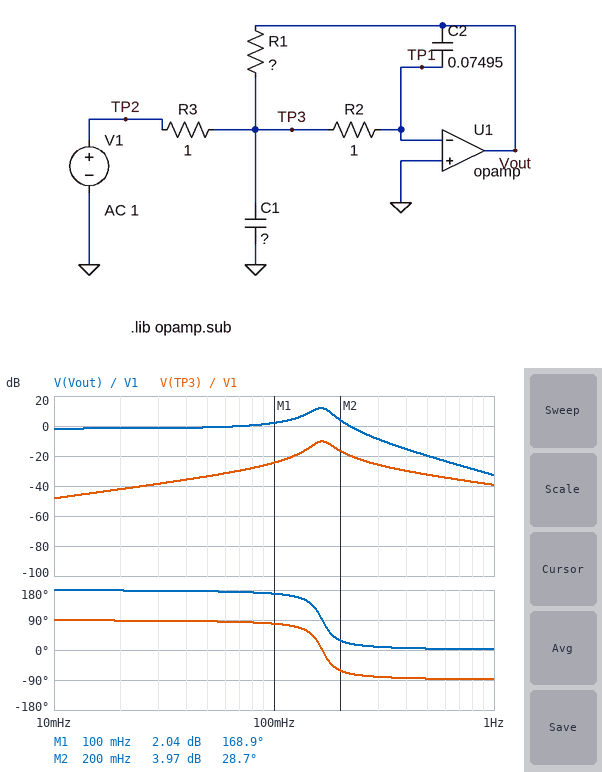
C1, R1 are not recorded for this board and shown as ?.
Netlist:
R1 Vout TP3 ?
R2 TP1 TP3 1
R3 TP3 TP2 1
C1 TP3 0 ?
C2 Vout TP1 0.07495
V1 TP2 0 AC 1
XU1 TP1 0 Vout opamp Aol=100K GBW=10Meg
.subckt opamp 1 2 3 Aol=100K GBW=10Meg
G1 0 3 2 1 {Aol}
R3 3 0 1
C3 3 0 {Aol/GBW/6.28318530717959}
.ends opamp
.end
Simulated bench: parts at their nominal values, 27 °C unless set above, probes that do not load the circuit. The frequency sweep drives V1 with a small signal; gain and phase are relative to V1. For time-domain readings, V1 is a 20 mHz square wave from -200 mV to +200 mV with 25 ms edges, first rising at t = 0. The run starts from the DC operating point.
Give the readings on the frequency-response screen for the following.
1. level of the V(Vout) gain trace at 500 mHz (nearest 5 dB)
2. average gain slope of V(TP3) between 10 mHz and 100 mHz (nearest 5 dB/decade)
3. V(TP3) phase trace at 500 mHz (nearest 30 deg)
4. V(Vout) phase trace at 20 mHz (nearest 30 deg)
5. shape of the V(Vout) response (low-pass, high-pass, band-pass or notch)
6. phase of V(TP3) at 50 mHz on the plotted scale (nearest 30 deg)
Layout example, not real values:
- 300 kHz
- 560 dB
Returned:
- -20 dB
- 25 dB/decade
- -90 deg
- 180 deg
- low-pass
- 90 deg
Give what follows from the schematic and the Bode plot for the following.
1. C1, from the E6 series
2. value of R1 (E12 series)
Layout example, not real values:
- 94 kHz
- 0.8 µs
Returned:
- 15 F
- 0.82 Ω
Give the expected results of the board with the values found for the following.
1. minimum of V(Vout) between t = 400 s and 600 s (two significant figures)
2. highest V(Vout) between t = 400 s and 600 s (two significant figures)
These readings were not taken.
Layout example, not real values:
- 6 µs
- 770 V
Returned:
- -390 mV
- 390 mV
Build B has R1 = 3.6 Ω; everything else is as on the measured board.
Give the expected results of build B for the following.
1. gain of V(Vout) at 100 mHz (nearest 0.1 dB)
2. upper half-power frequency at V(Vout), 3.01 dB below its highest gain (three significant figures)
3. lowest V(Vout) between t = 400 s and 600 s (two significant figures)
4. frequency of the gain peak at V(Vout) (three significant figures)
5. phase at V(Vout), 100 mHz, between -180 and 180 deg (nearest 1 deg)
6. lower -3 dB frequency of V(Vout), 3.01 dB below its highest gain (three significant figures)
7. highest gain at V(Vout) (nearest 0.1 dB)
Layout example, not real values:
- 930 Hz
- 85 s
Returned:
- 14.1 dB
- 88.6 mHz
- -1.5 V
- 77.2 mHz
- 33 deg
- 63.8 mHz
- 21.5 dB
